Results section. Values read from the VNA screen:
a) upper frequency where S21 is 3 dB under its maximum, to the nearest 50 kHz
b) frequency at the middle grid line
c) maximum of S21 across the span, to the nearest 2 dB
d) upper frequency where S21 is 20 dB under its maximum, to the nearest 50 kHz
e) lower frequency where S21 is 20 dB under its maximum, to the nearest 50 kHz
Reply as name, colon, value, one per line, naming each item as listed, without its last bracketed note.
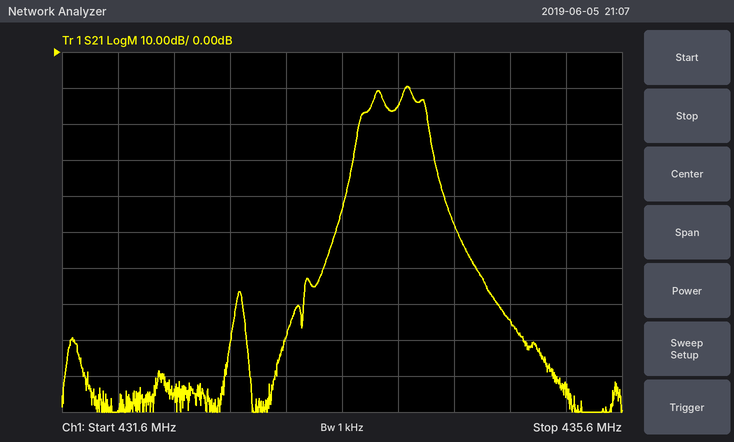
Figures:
upper frequency where S21 is 3 dB under its maximum, to the nearest 50 kHz: 434.10 MHz
frequency at the middle grid line: 433.6 MHz
maximum of S21 across the span, to the nearest 2 dB: -10 dB
upper frequency where S21 is 20 dB under its maximum, to the nearest 50 kHz: 434.25 MHz
lower frequency where S21 is 20 dB under its maximum, to the nearest 50 kHz: 433.70 MHz
